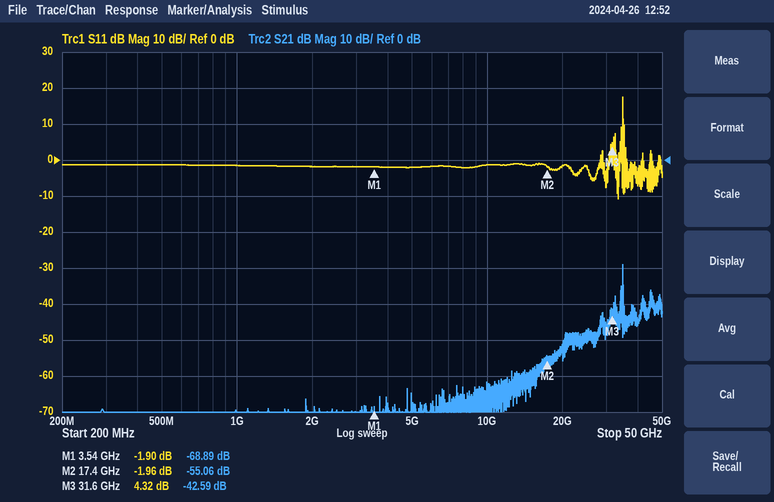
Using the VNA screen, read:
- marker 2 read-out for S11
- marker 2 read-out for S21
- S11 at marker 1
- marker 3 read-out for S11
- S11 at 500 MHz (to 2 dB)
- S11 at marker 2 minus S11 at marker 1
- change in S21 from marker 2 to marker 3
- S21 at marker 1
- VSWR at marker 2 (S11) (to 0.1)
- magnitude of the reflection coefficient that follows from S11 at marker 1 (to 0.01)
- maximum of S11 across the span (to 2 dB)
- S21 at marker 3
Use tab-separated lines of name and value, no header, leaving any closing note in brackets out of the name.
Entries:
marker 2 read-out for S11	-1.96 dB
marker 2 read-out for S21	-55.06 dB
S11 at marker 1	-1.90 dB
marker 3 read-out for S11	4.32 dB
S11 at 500 MHz	-2 dB
S11 at marker 2 minus S11 at marker 1	-0.06 dB
change in S21 from marker 2 to marker 3	12.47 dB
S21 at marker 1	-68.89 dB
VSWR at marker 2 (S11)	8.9
magnitude of the reflection coefficient that follows from S11 at marker 1	0.80
maximum of S11 across the span	18 dB
S21 at marker 3	-42.59 dB
